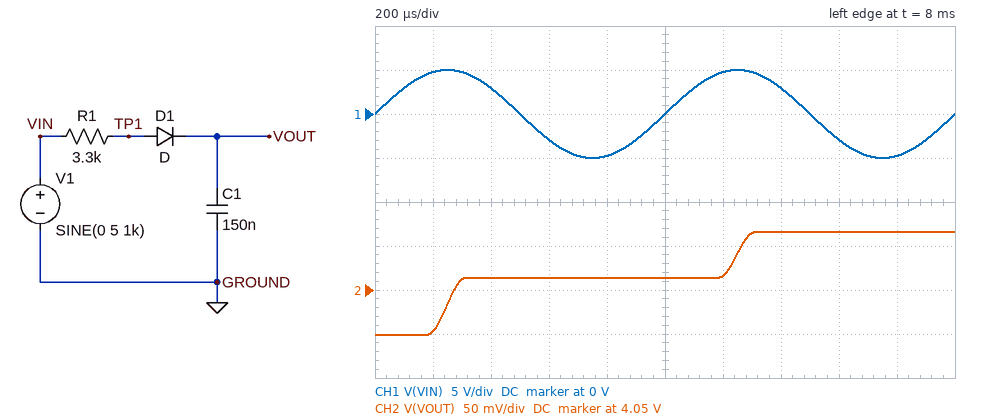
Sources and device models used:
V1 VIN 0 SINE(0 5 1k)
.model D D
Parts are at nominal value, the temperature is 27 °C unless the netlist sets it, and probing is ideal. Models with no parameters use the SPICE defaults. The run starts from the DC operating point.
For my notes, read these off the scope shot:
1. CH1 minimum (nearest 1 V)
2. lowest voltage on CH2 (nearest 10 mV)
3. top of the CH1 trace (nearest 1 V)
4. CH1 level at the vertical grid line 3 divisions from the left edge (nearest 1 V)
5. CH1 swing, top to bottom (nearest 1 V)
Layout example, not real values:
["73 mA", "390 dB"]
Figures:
["-5 V", "4.00 V", "5 V", "-3 V", "10 V"]
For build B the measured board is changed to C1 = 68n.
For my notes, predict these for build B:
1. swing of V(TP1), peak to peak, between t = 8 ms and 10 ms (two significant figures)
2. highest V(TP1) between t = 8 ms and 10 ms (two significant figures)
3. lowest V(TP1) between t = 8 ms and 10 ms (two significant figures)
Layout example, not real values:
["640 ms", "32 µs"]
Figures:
["9.9 V", "4.9 V", "-5.0 V"]
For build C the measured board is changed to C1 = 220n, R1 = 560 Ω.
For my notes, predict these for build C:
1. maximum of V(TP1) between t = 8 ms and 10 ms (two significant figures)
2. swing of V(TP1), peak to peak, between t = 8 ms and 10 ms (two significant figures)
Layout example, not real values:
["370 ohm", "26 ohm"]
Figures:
["5.0 V", "10 V"]
